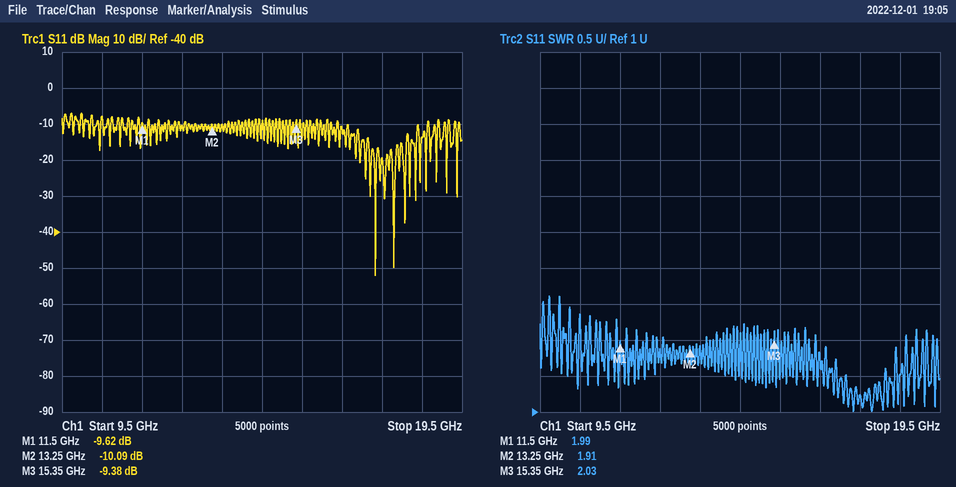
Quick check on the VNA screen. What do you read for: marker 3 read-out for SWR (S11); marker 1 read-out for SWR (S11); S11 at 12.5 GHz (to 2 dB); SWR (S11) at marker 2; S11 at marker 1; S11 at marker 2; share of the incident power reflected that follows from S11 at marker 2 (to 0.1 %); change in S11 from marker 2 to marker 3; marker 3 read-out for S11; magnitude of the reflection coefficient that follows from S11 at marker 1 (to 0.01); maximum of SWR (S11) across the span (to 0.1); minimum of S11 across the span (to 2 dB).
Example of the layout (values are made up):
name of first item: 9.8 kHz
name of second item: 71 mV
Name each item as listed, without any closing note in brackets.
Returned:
marker 3 read-out for SWR: 2.03
marker 1 read-out for SWR: 1.99
S11 at 12.5 GHz: -10 dB
SWR (S11) at marker 2: 1.91
S11 at marker 1: -9.62 dB
S11 at marker 2: -10.09 dB
share of the incident power reflected that follows from S11 at marker 2: 9.8 %
change in S11 from marker 2 to marker 3: 0.71 dB
marker 3 read-out for S11: -9.38 dB
magnitude of the reflection coefficient that follows from S11 at marker 1: 0.33
maximum of SWR (S11) across the span: 2.6
minimum of S11 across the span: -52 dB
